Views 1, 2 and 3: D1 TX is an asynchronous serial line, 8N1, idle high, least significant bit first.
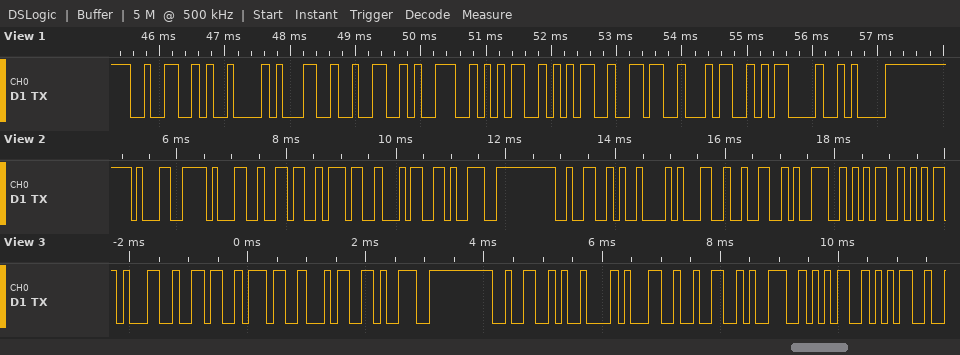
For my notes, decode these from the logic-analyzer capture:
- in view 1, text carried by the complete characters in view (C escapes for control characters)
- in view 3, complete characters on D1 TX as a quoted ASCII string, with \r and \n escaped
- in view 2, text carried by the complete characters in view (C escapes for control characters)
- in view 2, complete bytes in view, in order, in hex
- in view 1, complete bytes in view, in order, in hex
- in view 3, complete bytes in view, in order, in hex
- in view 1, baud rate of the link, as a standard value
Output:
"2\t1295564\r\n"
"167492\t12955"
"1167492\t1295"
31 31 36 37 34 39 32 09 31 32 39 35
32 09 31 32 39 35 35 36 34 0D 0A
0x31 0x36 0x37 0x34 0x39 0x32 0x09 0x31 0x32 0x39 0x35 0x35
9600 baud
